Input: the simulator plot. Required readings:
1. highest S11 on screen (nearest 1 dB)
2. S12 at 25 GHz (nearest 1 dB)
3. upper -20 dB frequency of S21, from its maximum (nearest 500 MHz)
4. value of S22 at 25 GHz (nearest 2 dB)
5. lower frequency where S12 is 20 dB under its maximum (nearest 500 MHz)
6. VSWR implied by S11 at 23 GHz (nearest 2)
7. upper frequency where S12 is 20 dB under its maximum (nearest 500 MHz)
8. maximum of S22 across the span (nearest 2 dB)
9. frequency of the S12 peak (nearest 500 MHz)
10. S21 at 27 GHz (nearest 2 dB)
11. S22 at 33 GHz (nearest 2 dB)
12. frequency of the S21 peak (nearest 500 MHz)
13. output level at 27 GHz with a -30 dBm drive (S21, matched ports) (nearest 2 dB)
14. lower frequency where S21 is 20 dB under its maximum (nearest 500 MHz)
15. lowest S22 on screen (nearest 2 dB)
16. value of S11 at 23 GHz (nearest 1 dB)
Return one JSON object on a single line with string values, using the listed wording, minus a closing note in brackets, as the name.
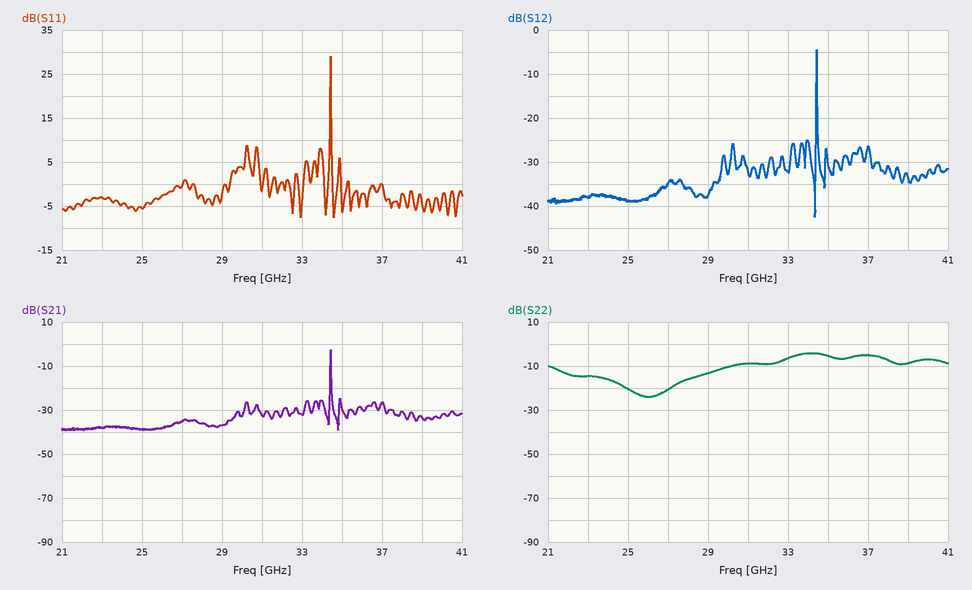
{"highest S11 on screen": "29 dB", "S12 at 25 GHz": "-39 dB", "upper -20 dB frequency of S21, from its maximum": "34.5 GHz", "value of S22 at 25 GHz": "-20 dB", "lower frequency where S12 is 20 dB under its maximum": "34.5 GHz", "VSWR implied by S11 at 23 GHz": "6", "upper frequency where S12 is 20 dB under its maximum": "34.5 GHz", "maximum of S22 across the span": "-4 dB", "frequency of the S12 peak": "34.5 GHz", "S21 at 27 GHz": "-36 dB", "S22 at 33 GHz": "-6 dB", "frequency of the S21 peak": "34.5 GHz", "output level at 27 GHz with a -30 dBm drive (S21, matched ports)": "-66 dBm", "lower frequency where S21 is 20 dB under its maximum": "34.5 GHz", "lowest S22 on screen": "-24 dB", "value of S11 at 23 GHz": "-3 dB"}
